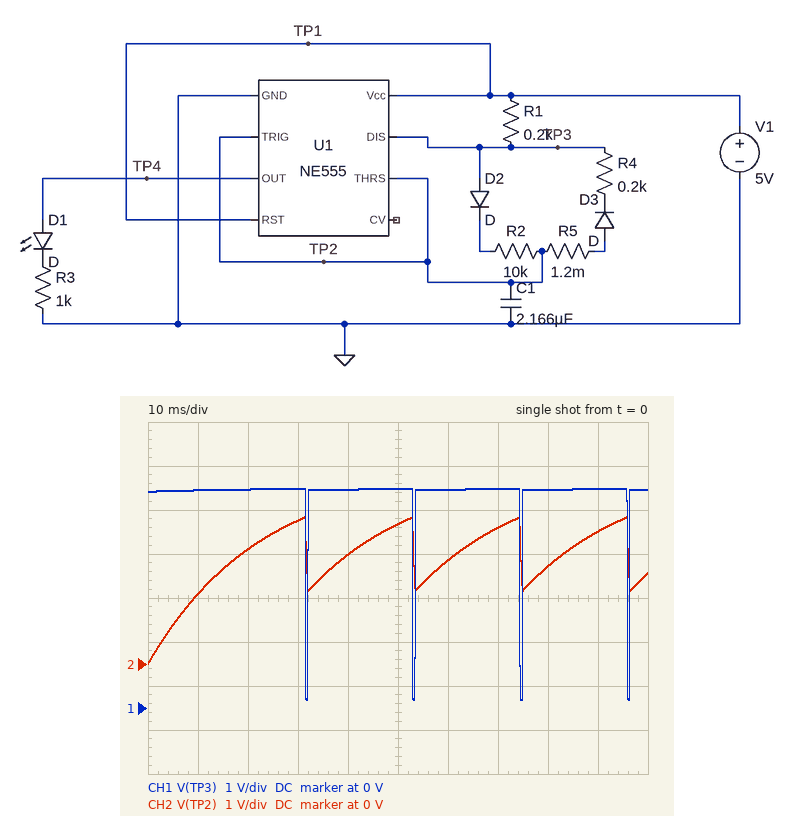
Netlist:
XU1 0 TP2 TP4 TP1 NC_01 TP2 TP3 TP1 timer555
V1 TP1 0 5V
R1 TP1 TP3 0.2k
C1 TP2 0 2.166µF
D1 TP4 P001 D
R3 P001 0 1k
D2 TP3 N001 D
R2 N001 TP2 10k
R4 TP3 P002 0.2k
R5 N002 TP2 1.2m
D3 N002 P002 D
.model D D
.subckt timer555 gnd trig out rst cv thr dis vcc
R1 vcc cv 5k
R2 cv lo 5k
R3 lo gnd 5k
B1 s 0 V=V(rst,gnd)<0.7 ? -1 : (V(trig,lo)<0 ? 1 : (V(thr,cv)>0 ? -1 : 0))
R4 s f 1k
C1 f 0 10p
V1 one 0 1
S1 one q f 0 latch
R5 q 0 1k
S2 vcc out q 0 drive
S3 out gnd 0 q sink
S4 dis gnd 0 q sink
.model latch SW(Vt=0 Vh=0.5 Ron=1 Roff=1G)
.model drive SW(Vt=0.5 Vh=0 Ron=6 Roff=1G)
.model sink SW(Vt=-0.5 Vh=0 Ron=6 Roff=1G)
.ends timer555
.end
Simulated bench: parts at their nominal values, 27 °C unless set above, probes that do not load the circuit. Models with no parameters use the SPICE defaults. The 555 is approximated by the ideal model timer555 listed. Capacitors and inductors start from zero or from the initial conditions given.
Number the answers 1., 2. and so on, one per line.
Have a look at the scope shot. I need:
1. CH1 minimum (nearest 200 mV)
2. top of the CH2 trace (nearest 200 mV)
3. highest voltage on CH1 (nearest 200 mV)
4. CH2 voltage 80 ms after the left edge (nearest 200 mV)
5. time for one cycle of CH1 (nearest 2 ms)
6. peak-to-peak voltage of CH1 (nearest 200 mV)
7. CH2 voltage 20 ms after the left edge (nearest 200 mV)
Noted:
1. 200 mV
2. 3.4 V
3. 5.0 V
4. 2.2 V
5. 22 ms
6. 4.8 V
7. 2.6 V
